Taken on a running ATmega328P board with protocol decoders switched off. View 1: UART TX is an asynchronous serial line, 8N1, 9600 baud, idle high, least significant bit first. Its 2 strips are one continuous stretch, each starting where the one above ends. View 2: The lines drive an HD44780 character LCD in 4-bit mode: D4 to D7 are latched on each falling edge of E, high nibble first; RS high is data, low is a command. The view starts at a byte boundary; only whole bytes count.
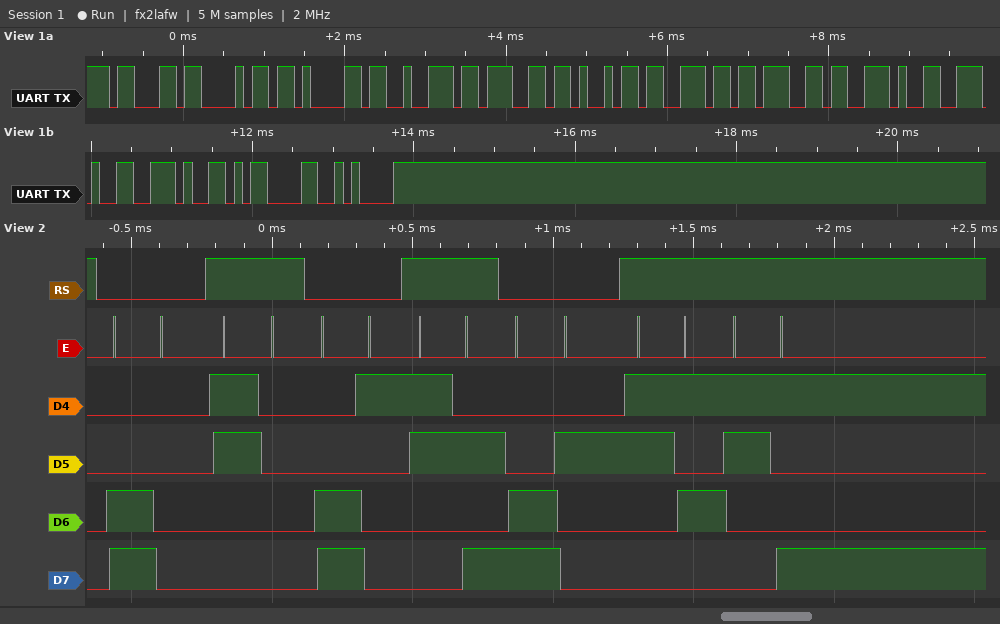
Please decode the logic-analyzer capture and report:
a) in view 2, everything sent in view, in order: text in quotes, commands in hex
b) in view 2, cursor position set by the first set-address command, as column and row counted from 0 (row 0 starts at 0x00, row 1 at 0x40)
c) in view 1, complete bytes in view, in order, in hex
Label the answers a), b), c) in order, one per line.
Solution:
a) 0xC0 "0" 0xC1 ":" 0xC2 "59"
b) column 0, row 1
c) 0x63 0x68 0x61 0x72 0x67 0x69 0x6E 0x67 0x2E 0x2E 0x2E 0x0D 0x0A
